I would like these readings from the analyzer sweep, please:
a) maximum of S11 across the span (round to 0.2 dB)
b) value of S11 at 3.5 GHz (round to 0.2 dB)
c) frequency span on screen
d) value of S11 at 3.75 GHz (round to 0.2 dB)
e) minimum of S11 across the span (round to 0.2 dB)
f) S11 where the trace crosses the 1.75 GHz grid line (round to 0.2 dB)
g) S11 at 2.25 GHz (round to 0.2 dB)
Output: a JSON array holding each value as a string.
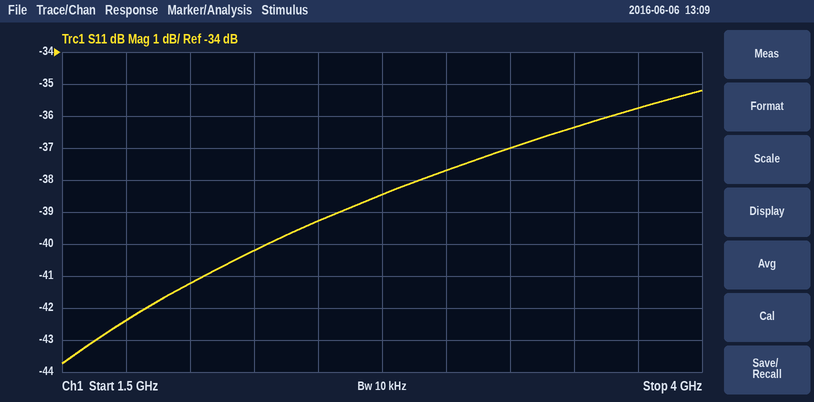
["-35.2 dB", "-36.4 dB", "2.5 GHz", "-35.8 dB", "-43.8 dB", "-42.4 dB", "-40.2 dB"]
